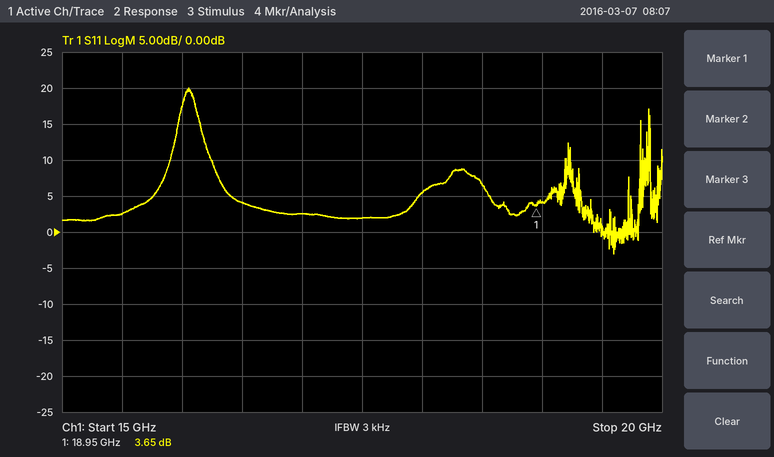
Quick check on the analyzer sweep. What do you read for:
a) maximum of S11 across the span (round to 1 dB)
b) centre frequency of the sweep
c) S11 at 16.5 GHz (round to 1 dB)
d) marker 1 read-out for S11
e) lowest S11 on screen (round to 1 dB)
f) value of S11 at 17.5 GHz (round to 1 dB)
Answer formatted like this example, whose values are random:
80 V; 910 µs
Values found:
20 dB; 17.5 GHz; 4 dB; 3.65 dB; -3 dB; 2 dB
